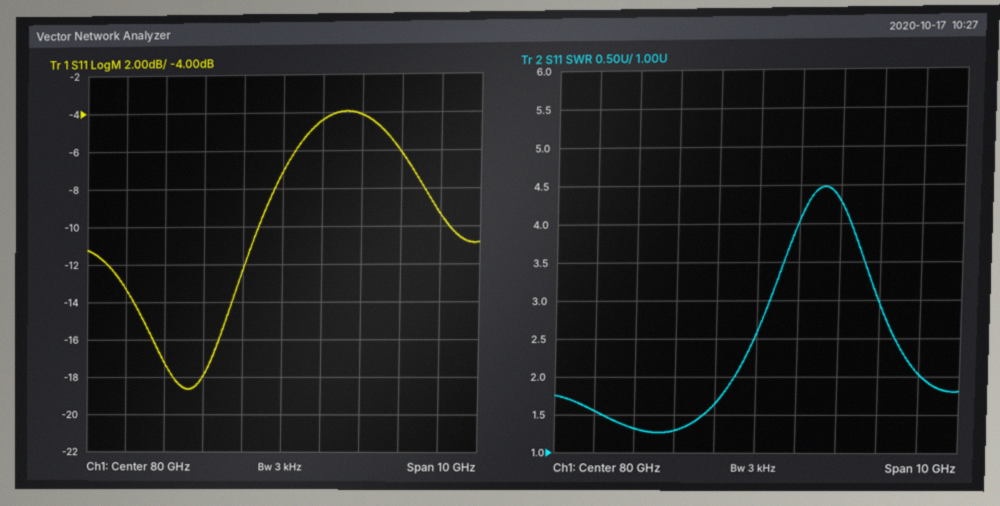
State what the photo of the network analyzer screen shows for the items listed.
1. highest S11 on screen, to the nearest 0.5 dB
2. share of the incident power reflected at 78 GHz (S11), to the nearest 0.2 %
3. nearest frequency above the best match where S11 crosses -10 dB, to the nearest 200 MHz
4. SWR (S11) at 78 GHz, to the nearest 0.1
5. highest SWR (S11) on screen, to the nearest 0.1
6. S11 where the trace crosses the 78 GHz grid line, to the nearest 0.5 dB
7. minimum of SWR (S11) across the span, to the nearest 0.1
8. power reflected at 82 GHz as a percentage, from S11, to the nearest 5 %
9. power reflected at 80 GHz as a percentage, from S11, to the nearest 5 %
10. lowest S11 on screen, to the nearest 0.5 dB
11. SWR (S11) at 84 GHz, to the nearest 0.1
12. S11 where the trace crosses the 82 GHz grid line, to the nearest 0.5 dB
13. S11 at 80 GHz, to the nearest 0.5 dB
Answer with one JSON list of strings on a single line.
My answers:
["-4.0 dB", "1.6 %", "79.4 GHz", "1.3", "4.5", "-18.0 dB", "1.3", "40 %", "20 %", "-18.5 dB", "2.0", "-4.0 dB", "-7.0 dB"]
